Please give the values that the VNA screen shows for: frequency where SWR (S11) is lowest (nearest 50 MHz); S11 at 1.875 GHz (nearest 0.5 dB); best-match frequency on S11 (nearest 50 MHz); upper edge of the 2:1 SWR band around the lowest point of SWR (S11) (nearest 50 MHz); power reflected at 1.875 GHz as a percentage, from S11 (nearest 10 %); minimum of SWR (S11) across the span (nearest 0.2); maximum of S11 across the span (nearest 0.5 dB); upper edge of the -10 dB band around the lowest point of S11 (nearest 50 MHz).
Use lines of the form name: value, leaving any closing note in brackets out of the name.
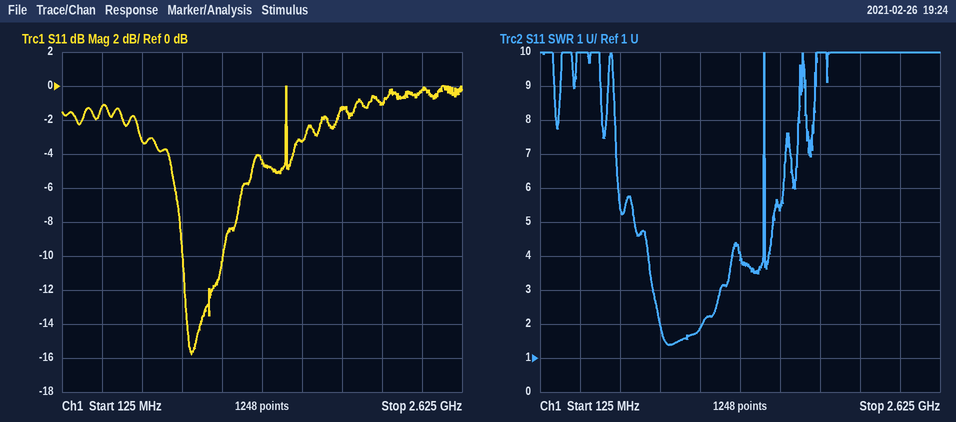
frequency where SWR (S11) is lowest: 950 MHz
S11 at 1.875 GHz: -1.5 dB
best-match frequency on S11: 950 MHz
upper edge of the 2:1 SWR band around the lowest point of SWR (S11): 1.15 GHz
power reflected at 1.875 GHz as a percentage, from S11: 70 %
minimum of SWR (S11) across the span: 1.4
maximum of S11 across the span: 0.0 dB
upper edge of the -10 dB band around the lowest point of S11: 1.15 GHz
